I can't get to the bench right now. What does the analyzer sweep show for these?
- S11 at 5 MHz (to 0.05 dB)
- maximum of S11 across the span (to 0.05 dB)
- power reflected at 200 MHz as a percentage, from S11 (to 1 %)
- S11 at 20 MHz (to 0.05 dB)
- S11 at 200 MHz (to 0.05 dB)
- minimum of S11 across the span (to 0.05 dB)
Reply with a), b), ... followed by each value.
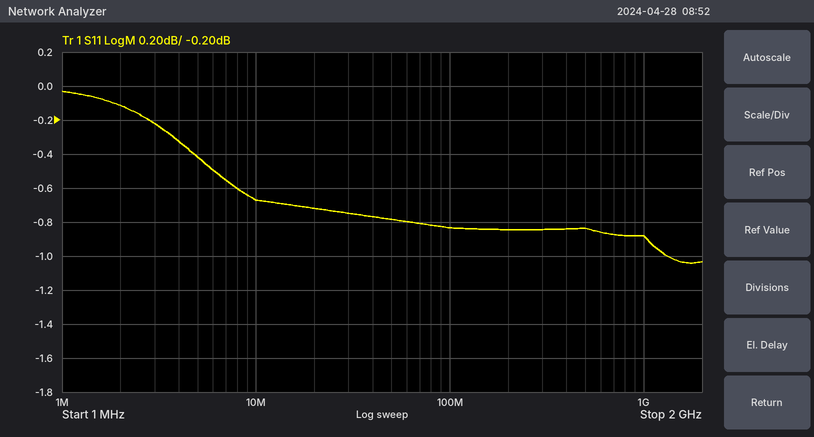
a) -0.40 dB
b) -0.05 dB
c) 82 %
d) -0.70 dB
e) -0.85 dB
f) -1.05 dB
